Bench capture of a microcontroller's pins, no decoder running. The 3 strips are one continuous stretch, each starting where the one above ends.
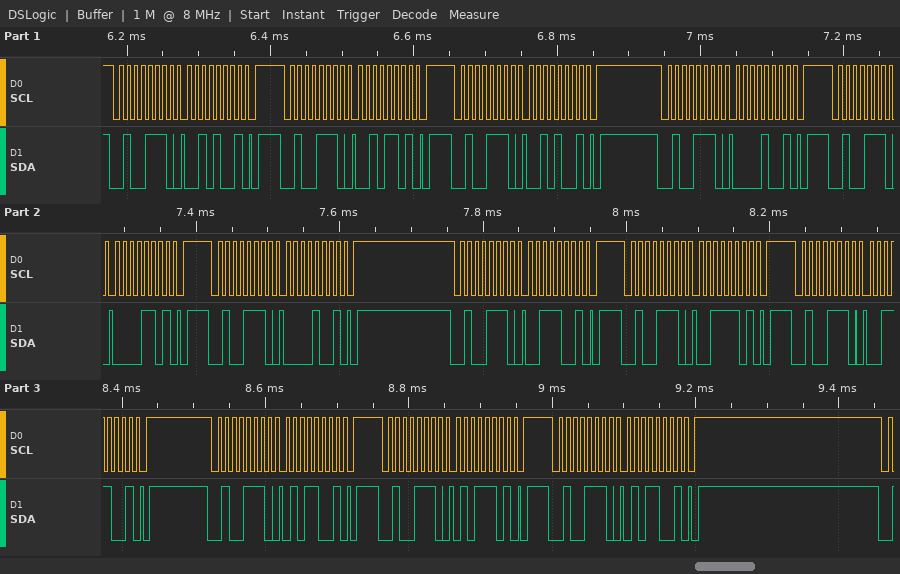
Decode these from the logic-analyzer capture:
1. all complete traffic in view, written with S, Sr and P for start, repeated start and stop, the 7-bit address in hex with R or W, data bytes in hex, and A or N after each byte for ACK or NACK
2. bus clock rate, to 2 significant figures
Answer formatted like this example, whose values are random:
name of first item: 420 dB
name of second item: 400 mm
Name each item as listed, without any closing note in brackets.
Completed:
all complete traffic in view, written with S, Sr and P for start, repeated start and stop, the 7-bit address in hex with R or W, data bytes in hex, and A or N after each byte for ACK or NACK: S 27W A 29 A P S 27W A 2D A P S 27W A 29 A P S 27W A 09 A P S 27W A 0D A P S 27W A 09 A P S 27W A 39 A P S 27W A 3D A P S 27W A 39 A P S 27W A 59 A P S 27W A 5D A P S 27W A 59 A P
bus clock rate, to 2 significant figures: 100 kHz
